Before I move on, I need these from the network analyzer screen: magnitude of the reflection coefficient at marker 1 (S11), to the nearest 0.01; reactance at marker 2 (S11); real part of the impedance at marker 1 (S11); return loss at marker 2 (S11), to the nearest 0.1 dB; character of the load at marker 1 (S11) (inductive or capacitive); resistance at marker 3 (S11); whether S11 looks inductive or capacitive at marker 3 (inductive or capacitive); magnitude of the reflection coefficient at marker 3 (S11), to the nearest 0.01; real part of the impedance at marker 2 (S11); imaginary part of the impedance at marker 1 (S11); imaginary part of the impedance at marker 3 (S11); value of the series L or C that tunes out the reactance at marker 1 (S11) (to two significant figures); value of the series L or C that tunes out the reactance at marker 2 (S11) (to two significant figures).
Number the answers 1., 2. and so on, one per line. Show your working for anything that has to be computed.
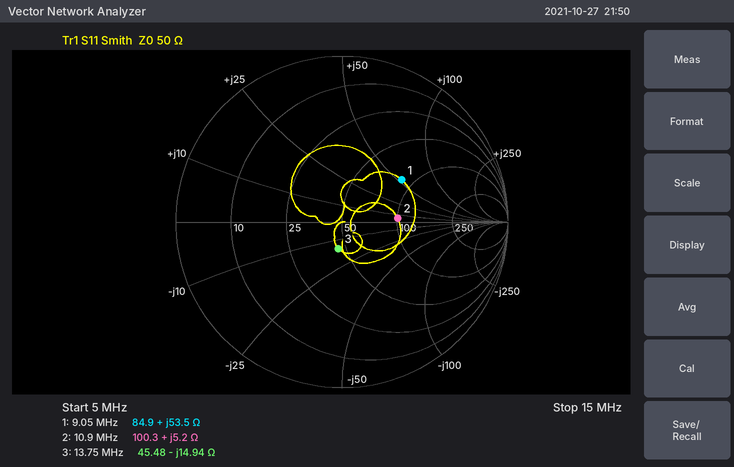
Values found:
1. 0.44
2. +5.2 Ω
3. 84.9 Ω
4. 9.5 dB
5. inductive
6. 45.48 Ω
7. capacitive
8. 0.16
9. 100.3 Ω
10. +53.5 Ω
11. -14.94 Ω
12. C = 1/(2π × 9.05 MHz × 53.5 Ω) ≈ 329 pF, so 330 pF to two significant figures
13. C = 1/(2π × 10.9 MHz × 5.2 Ω) ≈ 2.8 nF
